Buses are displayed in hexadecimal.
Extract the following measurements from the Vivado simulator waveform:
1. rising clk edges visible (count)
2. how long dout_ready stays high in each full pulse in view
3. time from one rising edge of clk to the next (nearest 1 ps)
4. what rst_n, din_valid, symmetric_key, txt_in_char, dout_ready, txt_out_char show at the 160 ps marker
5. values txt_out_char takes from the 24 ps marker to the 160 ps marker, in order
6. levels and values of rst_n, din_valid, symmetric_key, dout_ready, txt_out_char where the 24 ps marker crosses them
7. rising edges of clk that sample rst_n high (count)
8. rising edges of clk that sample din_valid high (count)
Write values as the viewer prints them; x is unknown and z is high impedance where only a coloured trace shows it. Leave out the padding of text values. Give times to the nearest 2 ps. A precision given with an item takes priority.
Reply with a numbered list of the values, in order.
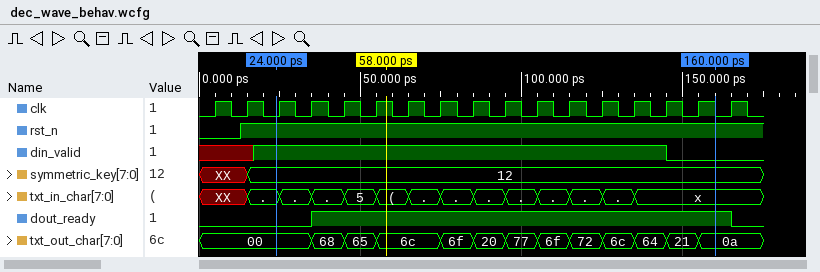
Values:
1. 17
2. 130 ps
3. 10 ps
4. rst_n=1, din_valid=0, symmetric_key=12, txt_in_char=x, dout_ready=1, txt_out_char=0a
5. 00, 68, 65, 6c, 6f, 20, 77, 6f, 72, 6c, 64, 21, 0a
6. rst_n=1, din_valid=1, symmetric_key=12, dout_ready=0, txt_out_char=00
7. 16
8. 13
